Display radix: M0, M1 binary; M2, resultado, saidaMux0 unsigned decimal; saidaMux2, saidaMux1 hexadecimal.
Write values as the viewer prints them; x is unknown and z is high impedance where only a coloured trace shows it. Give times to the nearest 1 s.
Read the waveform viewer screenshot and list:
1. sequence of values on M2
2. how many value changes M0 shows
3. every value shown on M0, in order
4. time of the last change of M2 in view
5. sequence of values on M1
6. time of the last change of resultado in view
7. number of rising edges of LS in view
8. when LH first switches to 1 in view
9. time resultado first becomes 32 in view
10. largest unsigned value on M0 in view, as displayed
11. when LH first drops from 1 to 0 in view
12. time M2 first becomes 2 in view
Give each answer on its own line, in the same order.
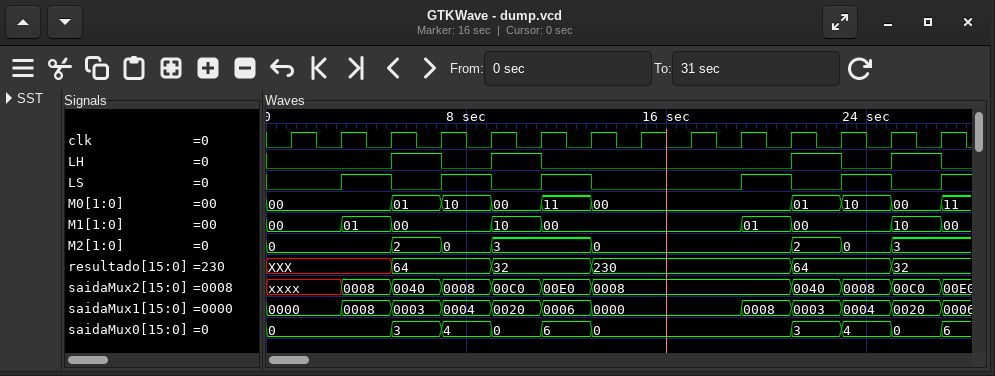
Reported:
0, 2, 0, 3, 0, 2, 0, 3
9
00, 01, 10, 00, 11, 00, 01, 10, 00, 11
25 s
00, 01, 00, 10, 00, 01, 00, 10, 00
25 s
6
5 s
9 s
11
7 s
5 s
